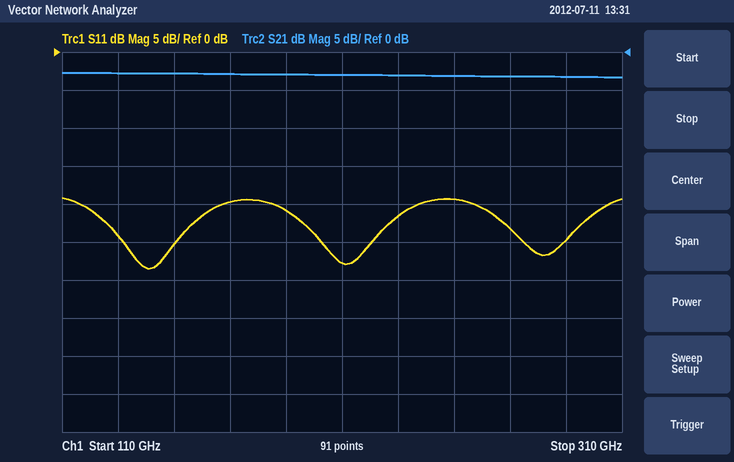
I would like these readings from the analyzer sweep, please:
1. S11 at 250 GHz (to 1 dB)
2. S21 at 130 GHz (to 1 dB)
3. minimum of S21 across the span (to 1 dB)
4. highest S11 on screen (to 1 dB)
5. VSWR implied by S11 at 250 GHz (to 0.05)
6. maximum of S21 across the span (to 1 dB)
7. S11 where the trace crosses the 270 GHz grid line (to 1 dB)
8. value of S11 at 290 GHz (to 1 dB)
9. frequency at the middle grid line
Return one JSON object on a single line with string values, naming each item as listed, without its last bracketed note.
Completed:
{"S11 at 250 GHz": "-19 dB", "S21 at 130 GHz": "-3 dB", "minimum of S21 across the span": "-3 dB", "highest S11 on screen": "-19 dB", "VSWR implied by S11 at 250 GHz": "1.25", "maximum of S21 across the span": "-3 dB", "S11 where the trace crosses the 270 GHz grid line": "-23 dB", "value of S11 at 290 GHz": "-25 dB", "frequency at the middle grid line": "210 GHz"}
